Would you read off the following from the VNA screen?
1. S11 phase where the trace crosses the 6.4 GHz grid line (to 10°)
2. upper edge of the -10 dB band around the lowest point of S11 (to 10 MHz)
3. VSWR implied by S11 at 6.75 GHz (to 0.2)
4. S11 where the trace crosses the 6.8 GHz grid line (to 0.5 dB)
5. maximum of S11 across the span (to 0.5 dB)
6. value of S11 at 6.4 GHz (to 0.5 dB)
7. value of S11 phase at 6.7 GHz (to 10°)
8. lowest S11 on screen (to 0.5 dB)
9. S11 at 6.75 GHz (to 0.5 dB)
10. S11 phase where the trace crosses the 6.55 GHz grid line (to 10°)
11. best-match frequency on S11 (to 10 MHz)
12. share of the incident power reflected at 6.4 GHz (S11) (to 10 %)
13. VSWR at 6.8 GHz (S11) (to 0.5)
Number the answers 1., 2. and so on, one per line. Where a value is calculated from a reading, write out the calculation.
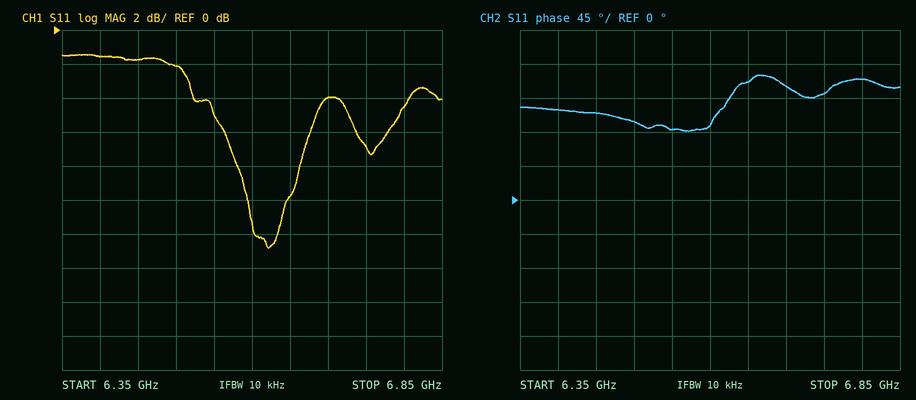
1. 120°
2. 6.65 GHz
3. |Γ| = 10^(-7/20) = 0.4467; VSWR = (1 + 0.4467)/(1 − 0.4467) ≈ 2.6
4. -4.5 dB
5. -1.5 dB
6. -1.5 dB
7. 150°
8. -13.0 dB
9. -7.0 dB
10. 90°
11. 6.62 GHz
12. 10^(-1.5/10) ≈ 70.8 %, so 70 % to the nearest 10 %
13. |Γ| = 10^(-4.5/20) = 0.5957; VSWR = (1 + 0.5957)/(1 − 0.5957) ≈ 4.0
